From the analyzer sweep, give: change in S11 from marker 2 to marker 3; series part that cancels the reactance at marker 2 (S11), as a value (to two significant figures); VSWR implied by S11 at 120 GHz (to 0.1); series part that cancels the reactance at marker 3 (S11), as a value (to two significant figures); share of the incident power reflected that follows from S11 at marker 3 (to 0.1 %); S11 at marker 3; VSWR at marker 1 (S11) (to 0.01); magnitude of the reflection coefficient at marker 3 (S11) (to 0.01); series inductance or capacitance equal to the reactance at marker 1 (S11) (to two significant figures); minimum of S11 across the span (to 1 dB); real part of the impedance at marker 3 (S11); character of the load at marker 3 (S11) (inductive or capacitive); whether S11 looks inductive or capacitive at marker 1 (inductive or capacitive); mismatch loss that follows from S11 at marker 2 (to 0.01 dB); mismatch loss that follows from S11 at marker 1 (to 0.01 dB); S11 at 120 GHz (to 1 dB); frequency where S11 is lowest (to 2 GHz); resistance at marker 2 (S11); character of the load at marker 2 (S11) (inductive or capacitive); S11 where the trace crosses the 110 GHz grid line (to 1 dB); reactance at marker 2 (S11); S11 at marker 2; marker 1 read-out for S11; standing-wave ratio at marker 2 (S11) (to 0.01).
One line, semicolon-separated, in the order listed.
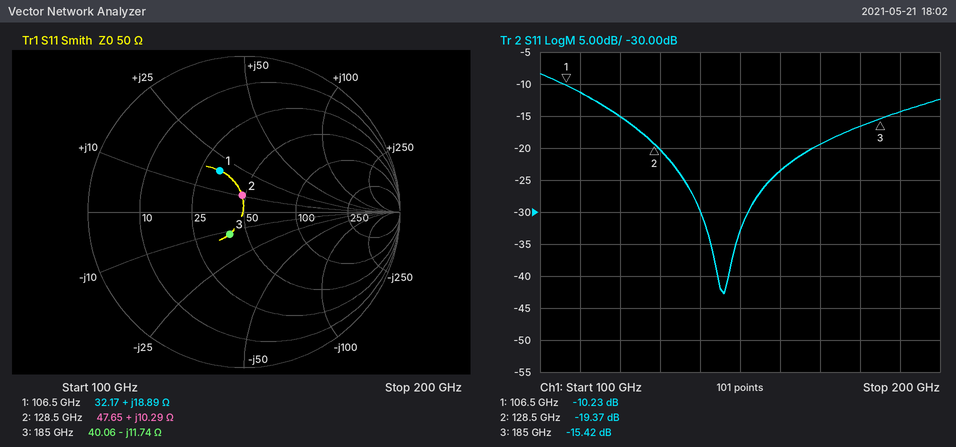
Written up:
3.95 dB; 120 fF; 1.4; 10 pH; 2.9 %; -15.42 dB; 1.89; 0.17; 28 pH; -43 dB; 40.06 Ω; capacitive; inductive; 0.05 dB; 0.43 dB; -15 dB; 146 GHz; 47.65 Ω; inductive; -11 dB; +10.29 Ω; -19.37 dB; -10.23 dB; 1.24
